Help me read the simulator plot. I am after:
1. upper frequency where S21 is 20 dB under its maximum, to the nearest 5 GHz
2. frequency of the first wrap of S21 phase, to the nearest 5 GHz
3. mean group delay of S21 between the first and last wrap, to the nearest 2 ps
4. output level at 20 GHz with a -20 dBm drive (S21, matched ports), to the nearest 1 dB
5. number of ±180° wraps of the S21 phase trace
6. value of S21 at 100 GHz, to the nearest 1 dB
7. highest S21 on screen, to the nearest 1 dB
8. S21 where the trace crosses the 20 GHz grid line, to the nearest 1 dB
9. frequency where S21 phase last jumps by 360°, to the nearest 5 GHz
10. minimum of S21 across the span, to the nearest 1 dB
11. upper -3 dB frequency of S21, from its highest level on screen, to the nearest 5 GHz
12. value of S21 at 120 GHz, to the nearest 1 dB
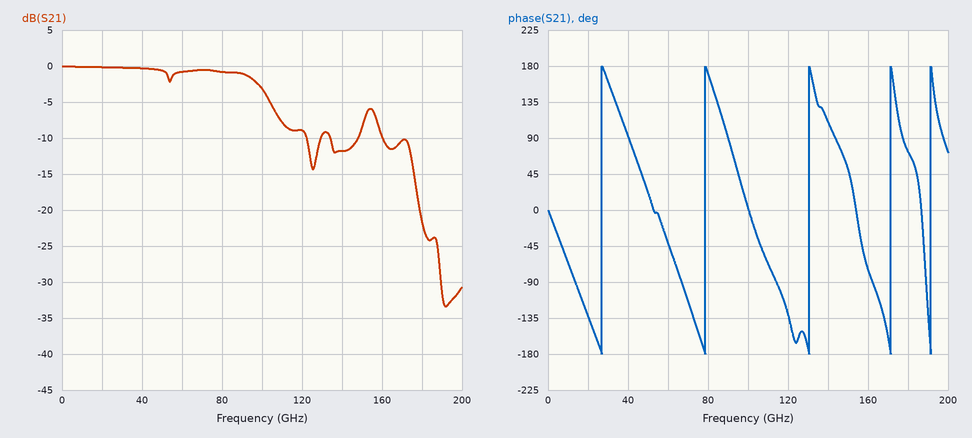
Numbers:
180 GHz
25 GHz
24 ps
-20 dBm
5
-3 dB
0 dB
0 dB
190 GHz
-33 dB
100 GHz
-9 dB
